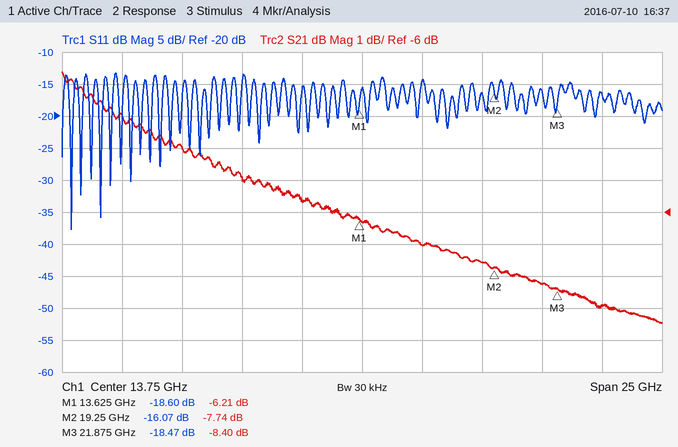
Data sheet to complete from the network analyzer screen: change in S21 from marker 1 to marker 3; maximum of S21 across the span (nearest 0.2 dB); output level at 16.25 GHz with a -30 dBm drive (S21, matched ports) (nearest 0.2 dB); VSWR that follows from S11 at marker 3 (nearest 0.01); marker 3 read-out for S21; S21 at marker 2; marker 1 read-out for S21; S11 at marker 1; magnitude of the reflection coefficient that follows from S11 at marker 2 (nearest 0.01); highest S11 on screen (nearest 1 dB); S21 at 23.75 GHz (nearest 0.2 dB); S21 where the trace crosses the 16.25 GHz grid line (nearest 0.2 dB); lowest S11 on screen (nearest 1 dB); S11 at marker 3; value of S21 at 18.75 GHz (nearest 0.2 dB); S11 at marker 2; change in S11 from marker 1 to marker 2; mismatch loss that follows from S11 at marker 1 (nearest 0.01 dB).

-2.19 dB
-1.6 dB
-37.0 dBm
1.27
-8.40 dB
-7.74 dB
-6.21 dB
-18.60 dB
0.16
-13 dB
-9.0 dB
-7.0 dB
-38 dB
-18.47 dB
-7.6 dB
-16.07 dB
2.53 dB
0.06 dB
